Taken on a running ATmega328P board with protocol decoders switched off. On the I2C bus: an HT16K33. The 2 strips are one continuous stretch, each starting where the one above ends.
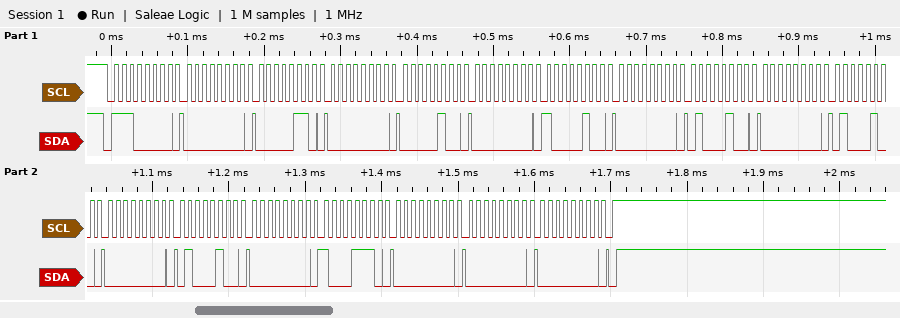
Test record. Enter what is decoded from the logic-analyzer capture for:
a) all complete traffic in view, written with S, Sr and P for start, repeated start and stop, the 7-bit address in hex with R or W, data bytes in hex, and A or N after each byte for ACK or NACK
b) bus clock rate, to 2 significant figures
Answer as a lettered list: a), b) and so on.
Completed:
a) S 70W A 00 A 06 A 00 A 04 A 00 A 84 A 00 A 44 A 00 A 44 A 00 A 44 A 00 A 8E A 00 A 00 A 00 A P
b) 100 kHz
